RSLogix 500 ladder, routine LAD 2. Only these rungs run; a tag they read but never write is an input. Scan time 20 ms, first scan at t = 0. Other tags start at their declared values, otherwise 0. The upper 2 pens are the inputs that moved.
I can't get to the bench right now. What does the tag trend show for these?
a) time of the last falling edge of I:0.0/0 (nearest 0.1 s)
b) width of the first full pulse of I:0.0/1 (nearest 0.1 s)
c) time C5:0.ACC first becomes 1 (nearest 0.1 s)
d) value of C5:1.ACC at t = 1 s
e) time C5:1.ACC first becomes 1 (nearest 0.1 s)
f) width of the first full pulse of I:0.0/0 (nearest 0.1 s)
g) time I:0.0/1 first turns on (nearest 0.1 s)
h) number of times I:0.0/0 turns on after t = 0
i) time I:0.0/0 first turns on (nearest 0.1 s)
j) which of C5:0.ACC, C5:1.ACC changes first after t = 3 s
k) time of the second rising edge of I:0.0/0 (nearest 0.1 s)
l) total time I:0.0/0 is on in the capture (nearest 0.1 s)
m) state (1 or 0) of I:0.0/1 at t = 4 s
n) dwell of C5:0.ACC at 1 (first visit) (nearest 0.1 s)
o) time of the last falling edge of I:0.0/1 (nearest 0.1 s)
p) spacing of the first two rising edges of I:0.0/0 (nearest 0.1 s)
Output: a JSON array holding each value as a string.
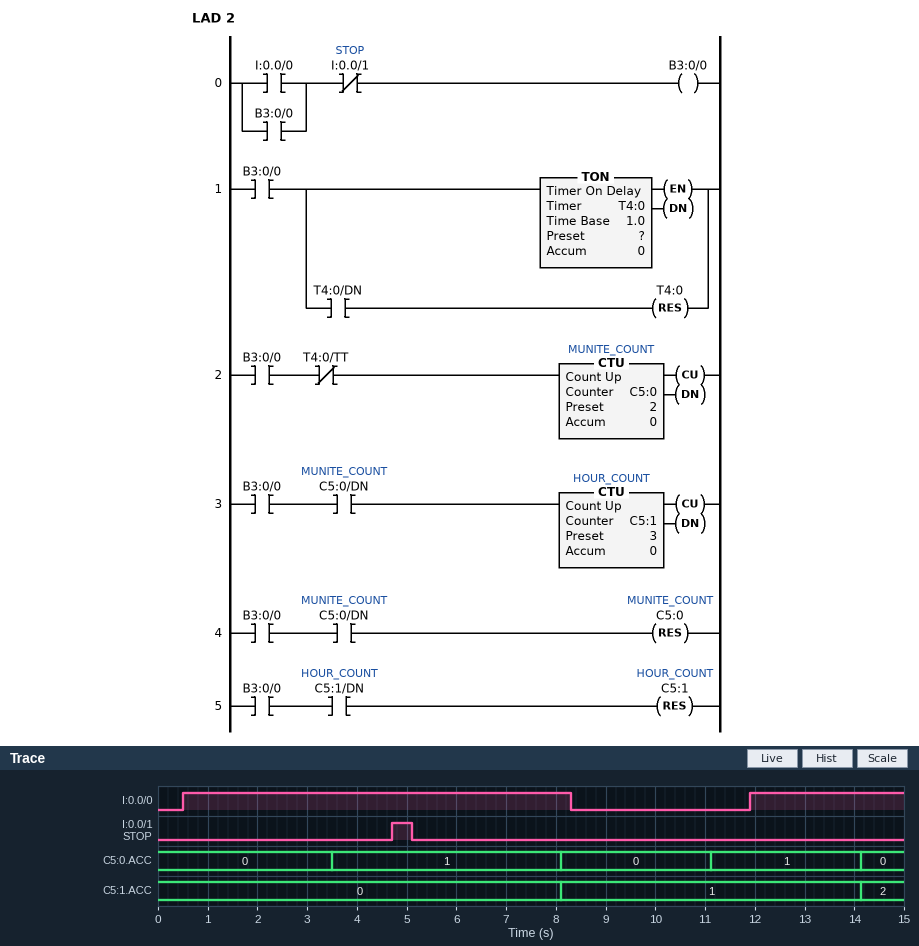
["8.3 s", "0.4 s", "3.5 s", "0", "8.1 s", "7.8 s", "4.7 s", "2", "0.5 s", "C5:0.ACC", "11.9 s", "10.9 s", "0", "4.6 s", "5.1 s", "11.4 s"]
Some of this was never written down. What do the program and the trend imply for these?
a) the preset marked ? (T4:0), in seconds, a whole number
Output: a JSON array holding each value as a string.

["3 s"]
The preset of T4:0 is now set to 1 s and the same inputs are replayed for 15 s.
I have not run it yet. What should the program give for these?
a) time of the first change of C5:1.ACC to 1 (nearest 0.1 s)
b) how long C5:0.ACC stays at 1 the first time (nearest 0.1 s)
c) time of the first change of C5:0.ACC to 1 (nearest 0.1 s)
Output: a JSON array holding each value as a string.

["2.5 s", "1.0 s", "1.5 s"]
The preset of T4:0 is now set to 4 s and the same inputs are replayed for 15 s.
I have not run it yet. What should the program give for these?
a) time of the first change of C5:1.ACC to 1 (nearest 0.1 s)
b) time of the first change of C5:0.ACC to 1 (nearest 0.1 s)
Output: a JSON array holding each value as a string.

["9.1 s", "4.5 s"]
